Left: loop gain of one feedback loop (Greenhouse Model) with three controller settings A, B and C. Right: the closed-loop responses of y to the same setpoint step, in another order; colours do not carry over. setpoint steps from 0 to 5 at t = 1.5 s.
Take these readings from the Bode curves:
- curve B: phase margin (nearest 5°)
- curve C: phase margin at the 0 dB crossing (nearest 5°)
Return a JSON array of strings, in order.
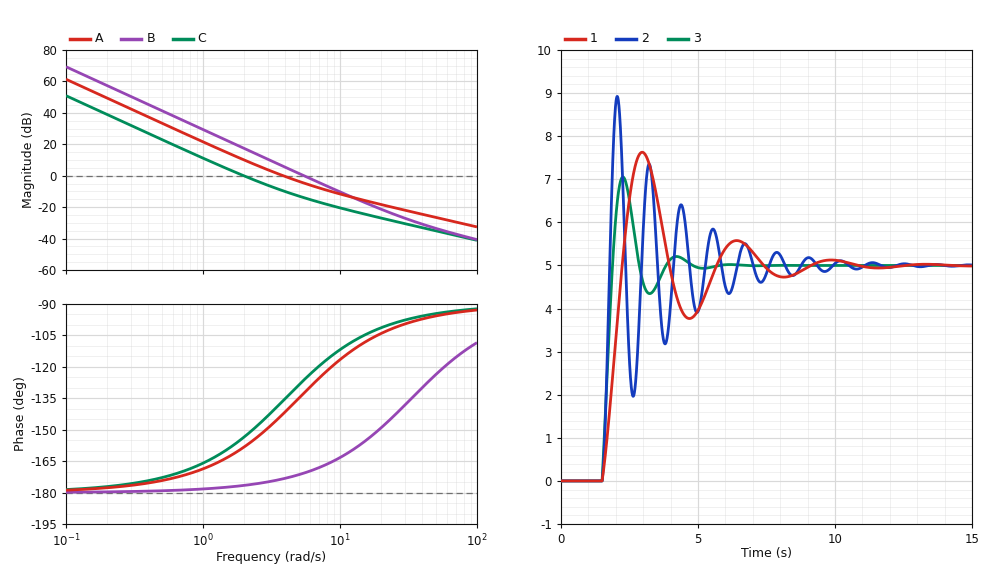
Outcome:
["10°", "25°"]
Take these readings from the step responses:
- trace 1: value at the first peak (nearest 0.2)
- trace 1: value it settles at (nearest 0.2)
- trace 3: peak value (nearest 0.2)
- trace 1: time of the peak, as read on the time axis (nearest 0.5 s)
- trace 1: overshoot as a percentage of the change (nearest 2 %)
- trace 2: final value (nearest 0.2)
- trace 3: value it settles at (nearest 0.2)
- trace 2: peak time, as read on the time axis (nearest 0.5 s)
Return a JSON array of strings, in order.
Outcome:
["7.6", "5.0", "7.0", "3.0 s", "52 %", "5.0", "5.0", "2.0 s"]
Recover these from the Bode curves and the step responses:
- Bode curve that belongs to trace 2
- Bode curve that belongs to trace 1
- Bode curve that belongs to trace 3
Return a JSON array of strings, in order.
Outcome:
["B", "C", "A"]
